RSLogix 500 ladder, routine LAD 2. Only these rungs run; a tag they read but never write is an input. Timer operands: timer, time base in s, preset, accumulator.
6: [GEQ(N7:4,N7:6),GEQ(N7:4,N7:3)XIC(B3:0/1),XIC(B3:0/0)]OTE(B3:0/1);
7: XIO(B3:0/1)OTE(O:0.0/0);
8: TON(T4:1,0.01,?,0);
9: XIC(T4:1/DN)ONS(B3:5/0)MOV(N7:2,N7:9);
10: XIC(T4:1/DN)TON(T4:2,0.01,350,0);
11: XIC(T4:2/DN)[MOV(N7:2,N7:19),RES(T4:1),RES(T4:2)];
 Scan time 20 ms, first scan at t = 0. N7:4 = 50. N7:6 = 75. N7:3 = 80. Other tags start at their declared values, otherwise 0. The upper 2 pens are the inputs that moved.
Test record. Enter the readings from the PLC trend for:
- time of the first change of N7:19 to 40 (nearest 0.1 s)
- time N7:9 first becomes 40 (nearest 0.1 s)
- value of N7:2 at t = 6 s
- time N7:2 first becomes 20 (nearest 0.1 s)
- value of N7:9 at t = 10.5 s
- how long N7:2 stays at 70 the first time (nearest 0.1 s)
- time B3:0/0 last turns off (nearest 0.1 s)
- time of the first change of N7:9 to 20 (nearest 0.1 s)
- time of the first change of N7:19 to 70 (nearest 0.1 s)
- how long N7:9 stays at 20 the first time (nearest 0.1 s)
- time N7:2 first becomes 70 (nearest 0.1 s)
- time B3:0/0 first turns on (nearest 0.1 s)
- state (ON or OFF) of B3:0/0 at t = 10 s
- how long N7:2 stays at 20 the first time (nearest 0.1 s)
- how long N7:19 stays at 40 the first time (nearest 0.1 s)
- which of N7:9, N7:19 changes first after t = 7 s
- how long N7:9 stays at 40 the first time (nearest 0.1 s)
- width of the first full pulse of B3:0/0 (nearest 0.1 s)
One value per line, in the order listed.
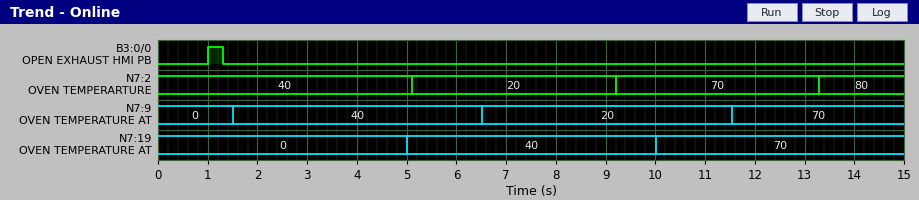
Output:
5.0 s
1.5 s
20
5.1 s
20
4.1 s
1.3 s
6.5 s
10.0 s
5.0 s
9.2 s
1.0 s
OFF
4.1 s
5.0 s
N7:19
5.0 s
0.3 s
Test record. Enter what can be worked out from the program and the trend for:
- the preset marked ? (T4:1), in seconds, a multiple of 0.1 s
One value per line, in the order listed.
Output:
1.5 s
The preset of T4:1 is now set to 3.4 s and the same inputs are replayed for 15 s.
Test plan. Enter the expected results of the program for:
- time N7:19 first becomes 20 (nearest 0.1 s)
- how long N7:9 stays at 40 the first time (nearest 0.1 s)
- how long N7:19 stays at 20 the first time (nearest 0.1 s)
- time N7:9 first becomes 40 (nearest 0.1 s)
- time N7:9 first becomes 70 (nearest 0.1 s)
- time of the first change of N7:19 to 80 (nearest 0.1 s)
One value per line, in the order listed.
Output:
6.9 s
6.9 s
6.9 s
3.4 s
10.3 s
13.8 s
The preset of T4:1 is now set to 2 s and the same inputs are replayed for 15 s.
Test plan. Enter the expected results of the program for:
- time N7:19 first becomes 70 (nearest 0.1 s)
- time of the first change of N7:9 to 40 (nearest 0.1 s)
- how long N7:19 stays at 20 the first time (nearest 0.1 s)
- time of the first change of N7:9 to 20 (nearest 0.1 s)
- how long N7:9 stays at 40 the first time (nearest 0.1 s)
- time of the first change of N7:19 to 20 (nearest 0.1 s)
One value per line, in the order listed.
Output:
11.0 s
2.0 s
5.5 s
7.5 s
5.5 s
5.5 s
